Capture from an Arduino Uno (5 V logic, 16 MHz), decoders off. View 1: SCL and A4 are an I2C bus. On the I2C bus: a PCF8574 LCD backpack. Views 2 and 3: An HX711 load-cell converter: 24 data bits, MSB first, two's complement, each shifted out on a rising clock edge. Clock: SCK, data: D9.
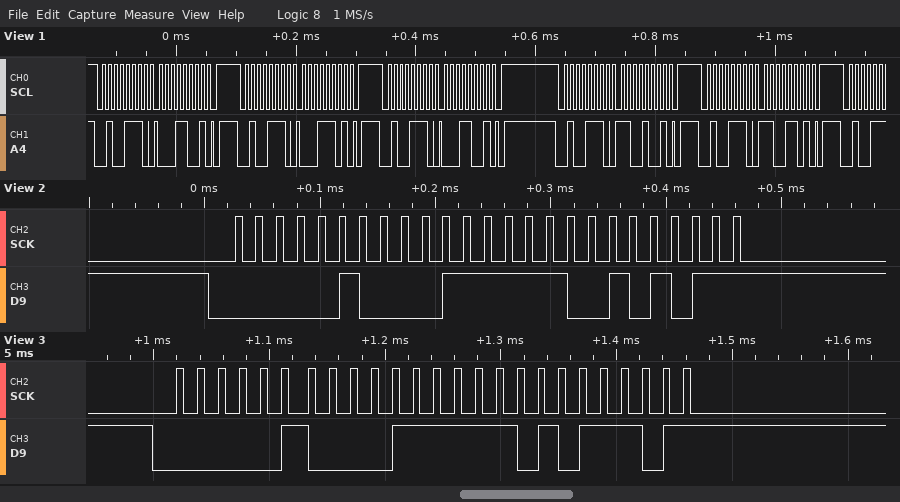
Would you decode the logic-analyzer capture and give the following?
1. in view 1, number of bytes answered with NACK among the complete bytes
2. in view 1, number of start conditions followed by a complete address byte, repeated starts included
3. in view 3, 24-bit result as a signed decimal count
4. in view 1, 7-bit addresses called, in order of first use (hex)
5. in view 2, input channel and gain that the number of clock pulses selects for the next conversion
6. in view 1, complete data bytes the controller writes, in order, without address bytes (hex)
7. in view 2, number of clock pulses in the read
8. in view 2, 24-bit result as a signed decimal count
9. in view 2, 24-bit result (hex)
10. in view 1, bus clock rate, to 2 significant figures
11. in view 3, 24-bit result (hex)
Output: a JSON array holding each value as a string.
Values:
["0", "5", "278365", "0x27", "channel A, gain 128", "19 1D 19 C9 CD", "25", "278315", "0x043F2B", "100 kHz", "0x043F5D"]
